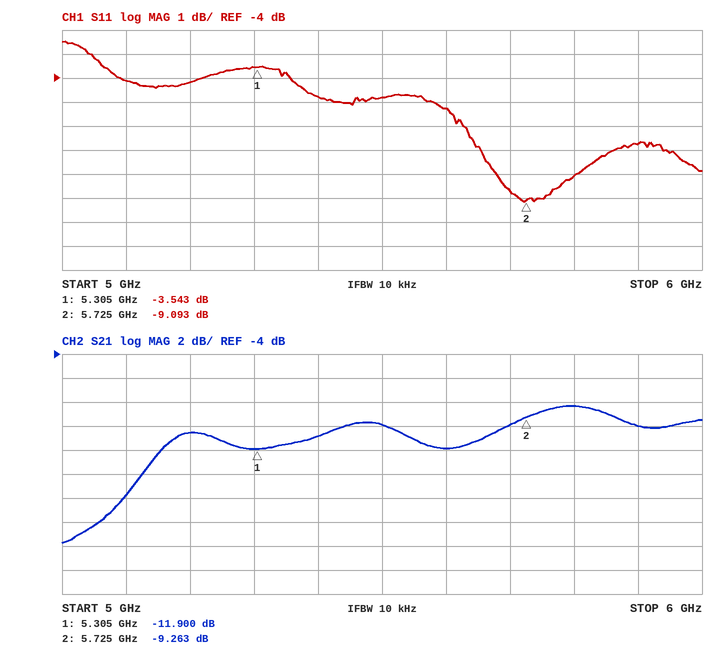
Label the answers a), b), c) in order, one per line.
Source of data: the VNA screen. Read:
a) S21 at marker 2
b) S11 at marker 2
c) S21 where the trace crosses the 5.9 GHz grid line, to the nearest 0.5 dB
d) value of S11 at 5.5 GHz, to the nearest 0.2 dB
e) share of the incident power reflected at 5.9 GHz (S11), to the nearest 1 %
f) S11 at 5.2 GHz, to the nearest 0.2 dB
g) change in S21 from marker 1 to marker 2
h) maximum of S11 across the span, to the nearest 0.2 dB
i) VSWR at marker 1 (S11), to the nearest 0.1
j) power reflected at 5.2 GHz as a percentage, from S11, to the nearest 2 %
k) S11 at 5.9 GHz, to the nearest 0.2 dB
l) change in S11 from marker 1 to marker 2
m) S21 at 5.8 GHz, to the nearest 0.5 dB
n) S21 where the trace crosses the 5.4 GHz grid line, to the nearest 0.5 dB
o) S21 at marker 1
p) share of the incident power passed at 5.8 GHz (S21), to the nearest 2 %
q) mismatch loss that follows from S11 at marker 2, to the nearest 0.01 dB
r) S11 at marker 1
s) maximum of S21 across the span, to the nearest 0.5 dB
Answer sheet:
a) -9.263 dB
b) -9.093 dB
c) -10.0 dB
d) -4.8 dB
e) 21 %
f) -4.2 dB
g) 2.637 dB
h) -2.4 dB
i) 5.0
j) 38 %
k) -6.8 dB
l) -5.550 dB
m) -8.5 dB
n) -11.0 dB
o) -11.900 dB
p) 14 %
q) 0.57 dB
r) -3.543 dB
s) -8.5 dB
